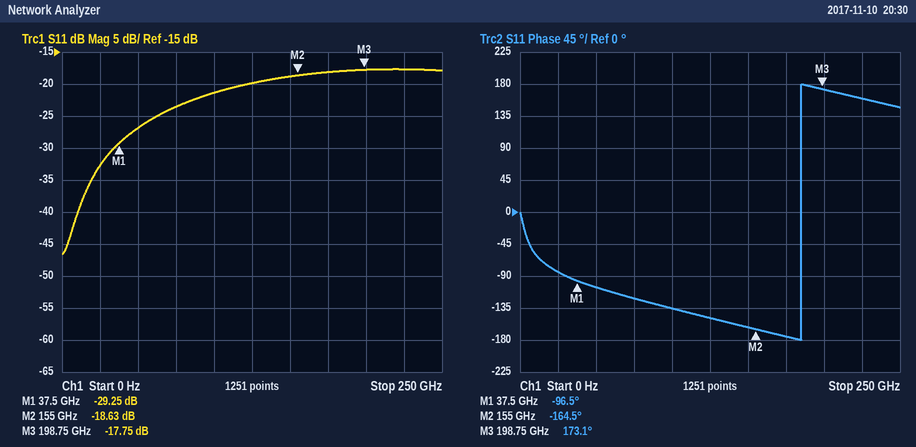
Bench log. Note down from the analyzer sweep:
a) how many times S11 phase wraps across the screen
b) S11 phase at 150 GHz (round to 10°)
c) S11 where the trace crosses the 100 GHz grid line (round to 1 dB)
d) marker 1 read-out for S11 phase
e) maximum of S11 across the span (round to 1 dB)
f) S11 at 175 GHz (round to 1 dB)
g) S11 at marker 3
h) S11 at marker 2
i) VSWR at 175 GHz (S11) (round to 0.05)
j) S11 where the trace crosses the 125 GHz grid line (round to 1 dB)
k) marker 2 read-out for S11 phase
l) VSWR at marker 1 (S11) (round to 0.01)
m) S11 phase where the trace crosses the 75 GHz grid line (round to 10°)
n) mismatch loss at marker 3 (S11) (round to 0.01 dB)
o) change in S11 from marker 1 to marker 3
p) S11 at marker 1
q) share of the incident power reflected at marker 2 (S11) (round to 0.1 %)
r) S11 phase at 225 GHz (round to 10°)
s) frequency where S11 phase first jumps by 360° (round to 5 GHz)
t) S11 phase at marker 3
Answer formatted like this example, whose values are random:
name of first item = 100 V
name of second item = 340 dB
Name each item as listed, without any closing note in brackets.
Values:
how many times S11 phase wraps across the screen = 1
S11 phase at 150 GHz = -160°
S11 where the trace crosses the 100 GHz grid line = -21 dB
marker 1 read-out for S11 phase = -96.5°
maximum of S11 across the span = -18 dB
S11 at 175 GHz = -18 dB
S11 at marker 3 = -17.75 dB
S11 at marker 2 = -18.63 dB
VSWR at 175 GHz (S11) = 1.30
S11 where the trace crosses the 125 GHz grid line = -20 dB
marker 2 read-out for S11 phase = -164.5°
VSWR at marker 1 (S11) = 1.07
S11 phase where the trace crosses the 75 GHz grid line = -120°
mismatch loss at marker 3 (S11) = 0.07 dB
change in S11 from marker 1 to marker 3 = 11.50 dB
S11 at marker 1 = -29.25 dB
share of the incident power reflected at marker 2 (S11) = 1.4 %
S11 phase at 225 GHz = 160°
frequency where S11 phase first jumps by 360° = 185 GHz
S11 phase at marker 3 = 173.1°
